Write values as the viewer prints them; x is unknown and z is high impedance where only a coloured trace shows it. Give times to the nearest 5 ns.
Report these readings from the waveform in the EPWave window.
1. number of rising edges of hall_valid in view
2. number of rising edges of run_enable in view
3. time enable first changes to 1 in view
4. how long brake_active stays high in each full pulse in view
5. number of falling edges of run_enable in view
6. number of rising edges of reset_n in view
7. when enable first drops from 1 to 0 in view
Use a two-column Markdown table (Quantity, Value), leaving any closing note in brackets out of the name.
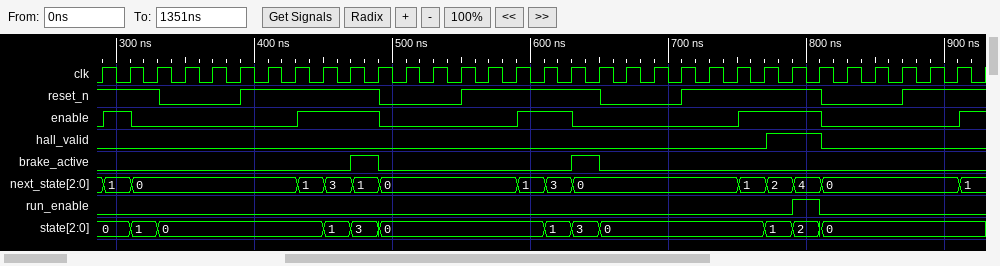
| Quantity | Value |
|---|---|
| number of rising edges of hall_valid in view | 1 |
| number of rising edges of run_enable in view | 1 |
| time enable first changes to 1 in view | 290 ns |
| how long brake_active stays high in each full pulse in view | 20 ns, 20 ns |
| number of falling edges of run_enable in view | 1 |
| number of rising edges of reset_n in view | 4 |
| when enable first drops from 1 to 0 in view | 310 ns |
